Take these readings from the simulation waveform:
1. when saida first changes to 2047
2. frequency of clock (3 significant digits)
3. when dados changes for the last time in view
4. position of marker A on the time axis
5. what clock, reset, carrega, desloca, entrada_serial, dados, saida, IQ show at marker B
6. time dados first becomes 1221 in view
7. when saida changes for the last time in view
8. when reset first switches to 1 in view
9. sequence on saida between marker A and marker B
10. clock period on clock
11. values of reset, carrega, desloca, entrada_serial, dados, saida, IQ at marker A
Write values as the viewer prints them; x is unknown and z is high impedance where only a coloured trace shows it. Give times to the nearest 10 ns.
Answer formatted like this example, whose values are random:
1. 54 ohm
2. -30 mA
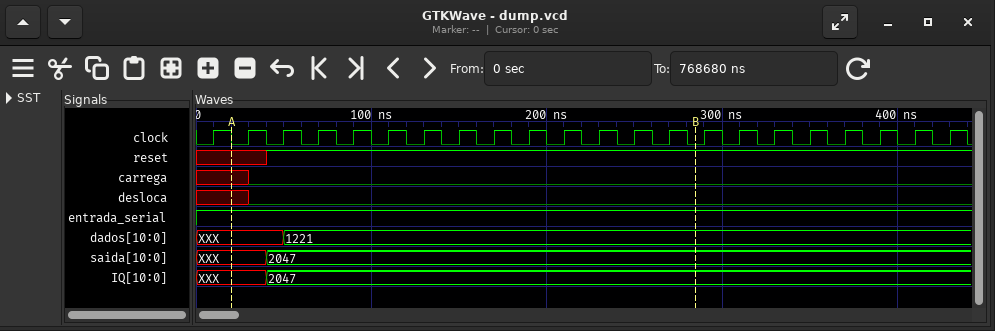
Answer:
1. 40 ns
2. 50.0 MHz
3. 50 ns
4. 20 ns
5. clock=0, reset=1, carrega=0, desloca=0, entrada_serial=1, dados=1221, saida=2047, IQ=2047
6. 50 ns
7. 40 ns
8. 40 ns
9. XXX, 2047
10. 20 ns
11. reset=x, carrega=x, desloca=x, entrada_serial=1, dados=XXX, saida=XXX, IQ=XXX
